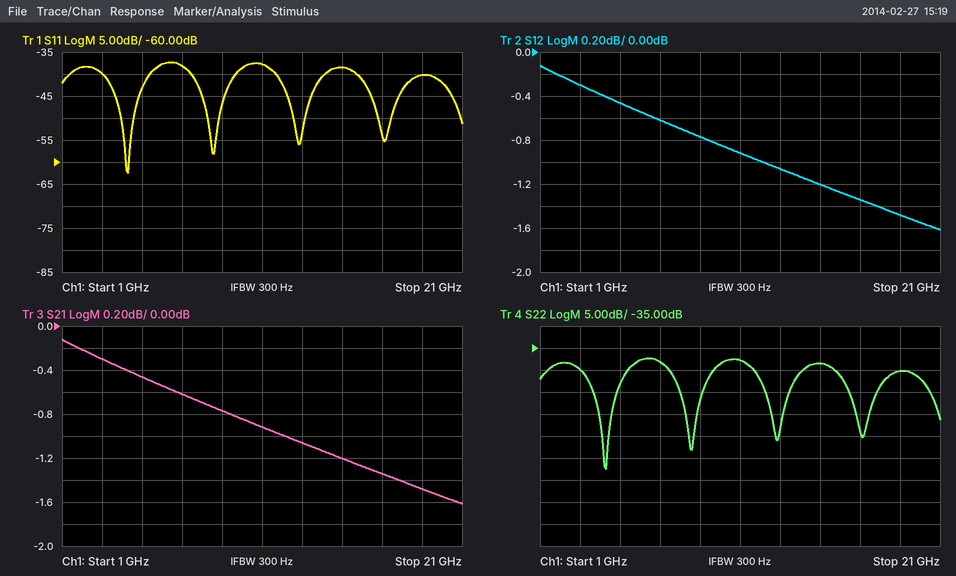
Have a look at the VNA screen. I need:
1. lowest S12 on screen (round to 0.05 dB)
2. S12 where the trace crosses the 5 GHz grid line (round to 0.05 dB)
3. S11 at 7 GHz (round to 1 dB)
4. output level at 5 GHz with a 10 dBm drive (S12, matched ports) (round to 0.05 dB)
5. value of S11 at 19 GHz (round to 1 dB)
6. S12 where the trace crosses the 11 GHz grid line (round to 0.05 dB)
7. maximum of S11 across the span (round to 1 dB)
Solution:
-1.60 dB
-0.45 dB
-38 dB
9.55 dBm
-40 dB
-0.90 dB
-37 dB
